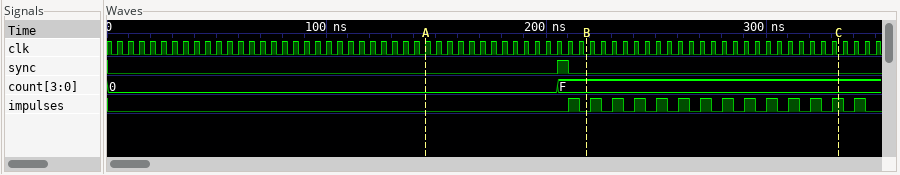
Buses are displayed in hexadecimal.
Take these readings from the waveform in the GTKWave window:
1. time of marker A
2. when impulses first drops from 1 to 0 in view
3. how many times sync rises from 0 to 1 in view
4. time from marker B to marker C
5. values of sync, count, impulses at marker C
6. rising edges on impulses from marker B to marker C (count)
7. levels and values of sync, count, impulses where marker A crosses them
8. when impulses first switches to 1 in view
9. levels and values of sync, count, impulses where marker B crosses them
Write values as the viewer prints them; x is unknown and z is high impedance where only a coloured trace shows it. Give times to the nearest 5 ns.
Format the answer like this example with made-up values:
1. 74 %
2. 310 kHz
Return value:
1. 145 ns
2. 215 ns
3. 1
4. 115 ns
5. sync=0, count=F, impulses=1
6. 12
7. sync=0, count=0, impulses=0
8. 210 ns
9. sync=0, count=F, impulses=0
